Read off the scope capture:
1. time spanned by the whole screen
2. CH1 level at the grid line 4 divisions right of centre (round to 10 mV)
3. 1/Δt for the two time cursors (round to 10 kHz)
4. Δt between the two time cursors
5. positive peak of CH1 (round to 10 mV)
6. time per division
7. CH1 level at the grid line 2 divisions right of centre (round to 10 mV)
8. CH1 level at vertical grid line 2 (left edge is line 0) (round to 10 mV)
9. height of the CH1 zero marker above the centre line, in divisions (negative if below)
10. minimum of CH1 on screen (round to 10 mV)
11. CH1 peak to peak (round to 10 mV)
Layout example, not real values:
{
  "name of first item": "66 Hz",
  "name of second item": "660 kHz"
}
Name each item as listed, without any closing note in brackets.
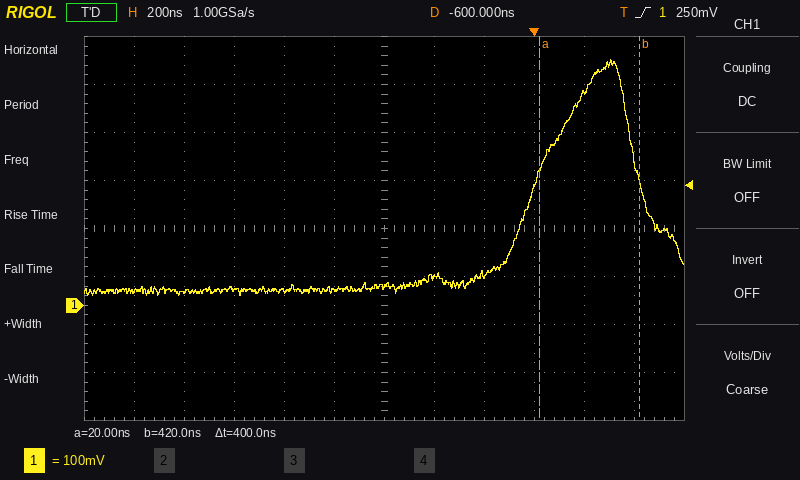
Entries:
{
  "time spanned by the whole screen": "2.4 µs",
  "CH1 level at the grid line 4 divisions right of centre": "440 mV",
  "1/Δt for the two time cursors": "2.50 MHz",
  "Δt between the two time cursors": "400 ns",
  "positive peak of CH1": "510 mV",
  "time per division": "200 ns",
  "CH1 level at the grid line 2 divisions right of centre": "60 mV",
  "CH1 level at vertical grid line 2 (left edge is line 0)": "30 mV",
  "height of the CH1 zero marker above the centre line, in divisions": "-1.6 div",
  "minimum of CH1 on screen": "20 mV",
  "CH1 peak to peak": "490 mV"
}
